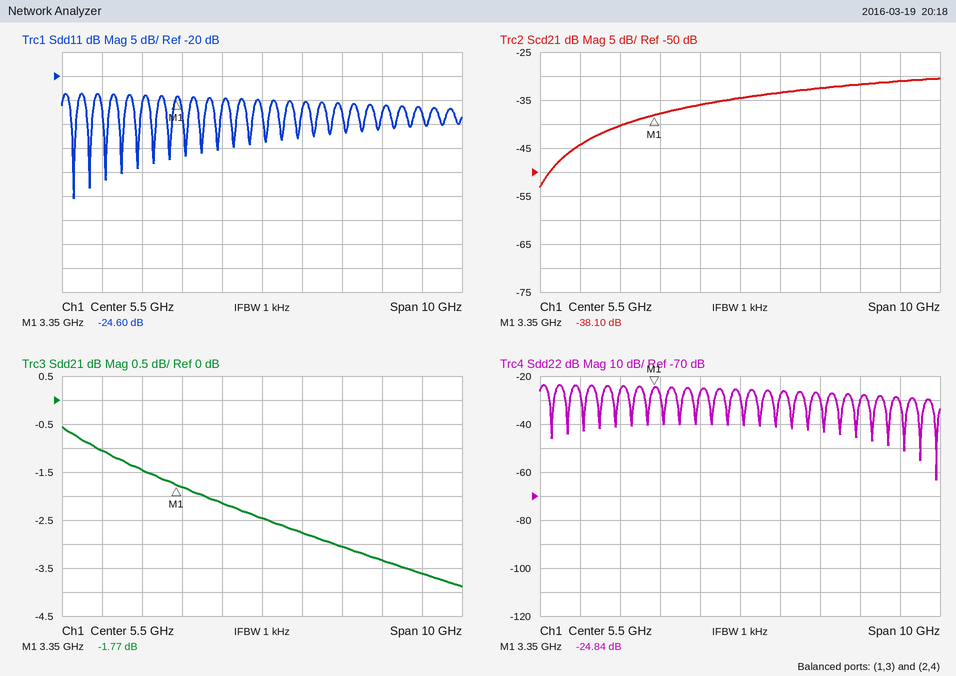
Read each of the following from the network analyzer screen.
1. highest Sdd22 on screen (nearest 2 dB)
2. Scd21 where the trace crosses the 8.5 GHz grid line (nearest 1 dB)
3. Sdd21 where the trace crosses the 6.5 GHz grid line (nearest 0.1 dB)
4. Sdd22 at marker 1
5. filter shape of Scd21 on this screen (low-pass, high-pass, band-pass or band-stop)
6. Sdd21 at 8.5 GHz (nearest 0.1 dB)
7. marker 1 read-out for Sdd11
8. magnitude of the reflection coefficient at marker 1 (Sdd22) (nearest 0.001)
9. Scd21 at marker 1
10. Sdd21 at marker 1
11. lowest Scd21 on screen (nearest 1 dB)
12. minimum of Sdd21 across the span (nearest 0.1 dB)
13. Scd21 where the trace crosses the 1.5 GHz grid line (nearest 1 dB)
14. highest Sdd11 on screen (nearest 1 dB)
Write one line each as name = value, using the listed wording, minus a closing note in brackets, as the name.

highest Sdd22 on screen = -24 dB
Scd21 where the trace crosses the 8.5 GHz grid line = -32 dB
Sdd21 where the trace crosses the 6.5 GHz grid line = -2.8 dB
Sdd22 at marker 1 = -24.84 dB
filter shape of Scd21 on this screen = high-pass
Sdd21 at 8.5 GHz = -3.3 dB
marker 1 read-out for Sdd11 = -24.60 dB
magnitude of the reflection coefficient at marker 1 (Sdd22) = 0.057
Scd21 at marker 1 = -38.10 dB
Sdd21 at marker 1 = -1.77 dB
lowest Scd21 on screen = -53 dB
minimum of Sdd21 across the span = -3.9 dB
Scd21 where the trace crosses the 1.5 GHz grid line = -44 dB
highest Sdd11 on screen = -24 dB
